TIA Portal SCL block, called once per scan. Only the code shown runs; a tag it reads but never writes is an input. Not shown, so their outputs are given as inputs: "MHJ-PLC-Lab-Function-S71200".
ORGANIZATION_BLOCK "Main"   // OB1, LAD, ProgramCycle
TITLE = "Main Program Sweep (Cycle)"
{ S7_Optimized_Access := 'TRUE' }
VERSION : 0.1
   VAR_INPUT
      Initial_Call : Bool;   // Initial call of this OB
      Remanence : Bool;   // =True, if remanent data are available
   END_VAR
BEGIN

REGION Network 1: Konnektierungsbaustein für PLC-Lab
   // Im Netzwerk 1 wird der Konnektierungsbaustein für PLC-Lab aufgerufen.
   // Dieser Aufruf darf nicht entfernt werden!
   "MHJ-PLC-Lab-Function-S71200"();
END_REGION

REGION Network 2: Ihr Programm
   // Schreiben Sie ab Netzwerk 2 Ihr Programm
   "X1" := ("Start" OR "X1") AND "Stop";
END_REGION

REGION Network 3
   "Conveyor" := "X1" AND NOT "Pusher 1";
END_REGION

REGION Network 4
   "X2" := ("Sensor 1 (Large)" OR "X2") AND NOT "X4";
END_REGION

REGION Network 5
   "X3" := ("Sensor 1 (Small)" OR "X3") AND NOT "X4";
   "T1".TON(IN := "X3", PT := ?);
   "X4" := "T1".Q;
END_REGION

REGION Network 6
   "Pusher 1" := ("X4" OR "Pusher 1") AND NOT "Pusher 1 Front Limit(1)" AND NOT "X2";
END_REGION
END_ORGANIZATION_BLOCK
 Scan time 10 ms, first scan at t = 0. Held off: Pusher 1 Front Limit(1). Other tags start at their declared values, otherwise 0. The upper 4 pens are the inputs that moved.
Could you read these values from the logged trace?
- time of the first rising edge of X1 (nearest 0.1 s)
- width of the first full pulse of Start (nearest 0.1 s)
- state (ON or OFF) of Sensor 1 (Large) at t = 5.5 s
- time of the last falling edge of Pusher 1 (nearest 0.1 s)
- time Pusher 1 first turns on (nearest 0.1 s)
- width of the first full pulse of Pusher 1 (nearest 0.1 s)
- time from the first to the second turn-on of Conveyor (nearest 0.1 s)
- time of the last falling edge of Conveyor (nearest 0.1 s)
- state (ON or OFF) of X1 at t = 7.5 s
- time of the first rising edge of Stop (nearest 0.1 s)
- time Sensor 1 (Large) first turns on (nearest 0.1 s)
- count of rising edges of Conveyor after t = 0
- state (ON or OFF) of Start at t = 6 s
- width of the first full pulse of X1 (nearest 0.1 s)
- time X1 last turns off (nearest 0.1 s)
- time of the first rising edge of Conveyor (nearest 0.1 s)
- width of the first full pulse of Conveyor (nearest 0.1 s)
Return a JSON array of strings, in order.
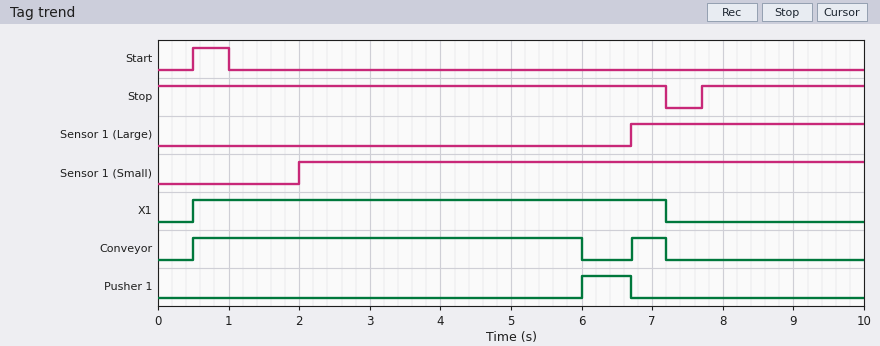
["0.5 s", "0.5 s", "OFF", "6.7 s", "6.0 s", "0.7 s", "6.2 s", "7.2 s", "OFF", "7.7 s", "6.7 s", "2", "OFF", "6.7 s", "7.2 s", "0.5 s", "5.5 s"]
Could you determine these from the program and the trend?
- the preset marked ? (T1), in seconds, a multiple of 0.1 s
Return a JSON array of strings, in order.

["4.0 s"]
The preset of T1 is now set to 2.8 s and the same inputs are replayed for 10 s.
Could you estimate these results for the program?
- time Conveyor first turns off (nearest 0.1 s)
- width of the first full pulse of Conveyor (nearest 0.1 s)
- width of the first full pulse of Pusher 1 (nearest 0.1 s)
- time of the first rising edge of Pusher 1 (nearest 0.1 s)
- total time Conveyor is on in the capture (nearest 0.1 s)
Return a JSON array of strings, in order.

["4.8 s", "4.3 s", "1.9 s", "4.8 s", "4.8 s"]
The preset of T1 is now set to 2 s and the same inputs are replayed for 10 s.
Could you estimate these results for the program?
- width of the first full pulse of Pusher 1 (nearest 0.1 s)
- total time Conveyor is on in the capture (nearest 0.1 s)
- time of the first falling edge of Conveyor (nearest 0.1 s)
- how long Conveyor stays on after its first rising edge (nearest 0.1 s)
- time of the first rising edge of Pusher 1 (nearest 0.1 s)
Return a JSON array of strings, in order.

["2.7 s", "4.0 s", "4.0 s", "3.5 s", "4.0 s"]
